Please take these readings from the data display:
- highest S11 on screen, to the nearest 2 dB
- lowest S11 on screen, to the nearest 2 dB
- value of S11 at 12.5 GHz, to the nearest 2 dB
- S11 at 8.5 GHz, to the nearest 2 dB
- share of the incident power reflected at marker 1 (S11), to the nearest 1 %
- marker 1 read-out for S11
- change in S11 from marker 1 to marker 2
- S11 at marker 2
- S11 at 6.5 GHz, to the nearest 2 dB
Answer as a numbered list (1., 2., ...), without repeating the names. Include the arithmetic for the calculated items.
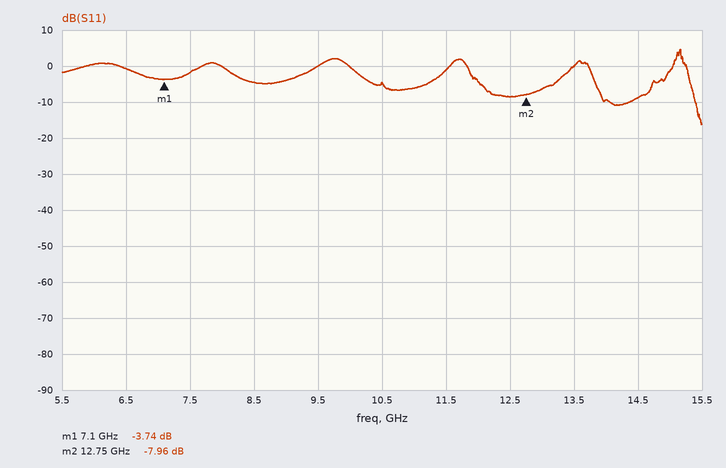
1. 4 dB
2. -16 dB
3. -8 dB
4. -4 dB
5. 10^(-3.74/10) ≈ 42 %
6. -3.74 dB
7. -7.96 − (-3.74) = -4.22 dB
8. -7.96 dB
9. 0 dB
